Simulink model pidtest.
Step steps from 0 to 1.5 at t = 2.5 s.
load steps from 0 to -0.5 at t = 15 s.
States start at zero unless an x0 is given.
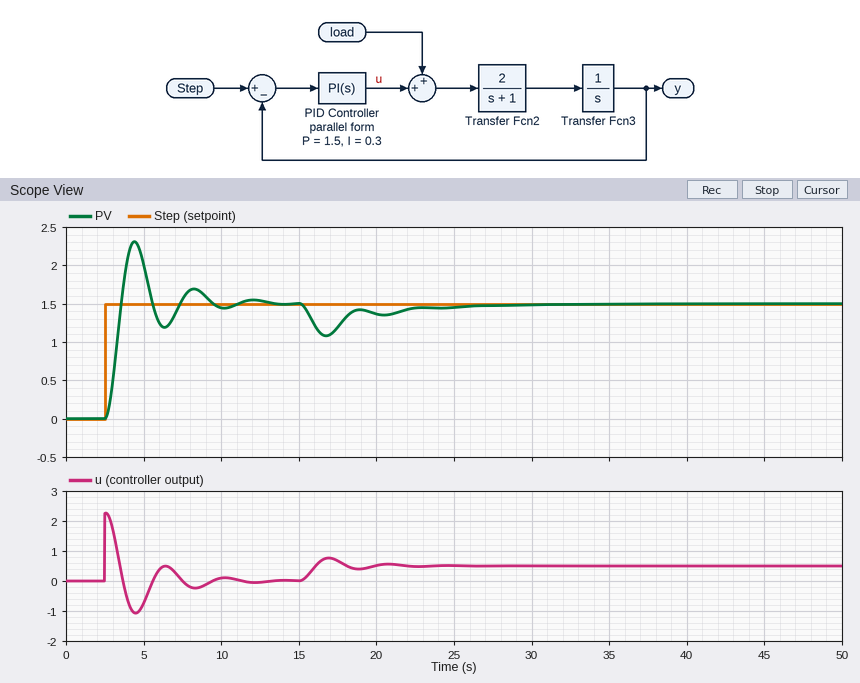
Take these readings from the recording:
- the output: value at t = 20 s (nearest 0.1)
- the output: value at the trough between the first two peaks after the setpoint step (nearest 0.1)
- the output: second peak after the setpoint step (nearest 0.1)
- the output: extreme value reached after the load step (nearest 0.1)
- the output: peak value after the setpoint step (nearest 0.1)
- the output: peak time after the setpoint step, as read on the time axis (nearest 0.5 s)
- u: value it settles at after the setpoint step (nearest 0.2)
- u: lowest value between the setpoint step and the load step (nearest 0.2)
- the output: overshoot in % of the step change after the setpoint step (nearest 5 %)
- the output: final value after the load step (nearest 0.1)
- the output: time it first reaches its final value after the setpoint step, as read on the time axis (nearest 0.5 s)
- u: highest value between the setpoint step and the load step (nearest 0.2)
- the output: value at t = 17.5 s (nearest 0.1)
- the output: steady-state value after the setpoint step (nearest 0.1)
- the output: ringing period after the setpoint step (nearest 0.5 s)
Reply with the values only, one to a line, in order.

1.4
1.2
1.7
1.1
2.3
4.5 s
0.0
-1.0
55 %
1.5
3.5 s
2.2
1.2
1.5
4.0 s
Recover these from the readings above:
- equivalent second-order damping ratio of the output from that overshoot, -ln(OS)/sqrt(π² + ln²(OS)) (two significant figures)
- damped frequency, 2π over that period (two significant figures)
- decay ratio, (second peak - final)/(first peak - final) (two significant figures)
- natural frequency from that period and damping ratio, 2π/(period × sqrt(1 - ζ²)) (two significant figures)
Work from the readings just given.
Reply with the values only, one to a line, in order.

0.19
1.6 rad/s
0.25
1.6 rad/s
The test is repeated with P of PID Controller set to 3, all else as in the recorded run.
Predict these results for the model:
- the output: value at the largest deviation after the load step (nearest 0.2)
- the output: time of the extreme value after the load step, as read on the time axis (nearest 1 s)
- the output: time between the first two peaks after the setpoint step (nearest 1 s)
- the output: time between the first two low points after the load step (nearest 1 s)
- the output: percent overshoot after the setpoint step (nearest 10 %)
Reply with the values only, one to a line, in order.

1.2
16 s
3 s
3 s
60 %
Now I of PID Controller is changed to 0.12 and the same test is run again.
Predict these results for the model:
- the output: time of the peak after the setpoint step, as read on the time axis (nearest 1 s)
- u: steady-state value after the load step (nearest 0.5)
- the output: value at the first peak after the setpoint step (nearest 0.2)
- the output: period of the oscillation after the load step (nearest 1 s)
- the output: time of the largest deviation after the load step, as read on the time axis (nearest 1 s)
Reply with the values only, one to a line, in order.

4 s
0.5
2.2
4 s
17 s
